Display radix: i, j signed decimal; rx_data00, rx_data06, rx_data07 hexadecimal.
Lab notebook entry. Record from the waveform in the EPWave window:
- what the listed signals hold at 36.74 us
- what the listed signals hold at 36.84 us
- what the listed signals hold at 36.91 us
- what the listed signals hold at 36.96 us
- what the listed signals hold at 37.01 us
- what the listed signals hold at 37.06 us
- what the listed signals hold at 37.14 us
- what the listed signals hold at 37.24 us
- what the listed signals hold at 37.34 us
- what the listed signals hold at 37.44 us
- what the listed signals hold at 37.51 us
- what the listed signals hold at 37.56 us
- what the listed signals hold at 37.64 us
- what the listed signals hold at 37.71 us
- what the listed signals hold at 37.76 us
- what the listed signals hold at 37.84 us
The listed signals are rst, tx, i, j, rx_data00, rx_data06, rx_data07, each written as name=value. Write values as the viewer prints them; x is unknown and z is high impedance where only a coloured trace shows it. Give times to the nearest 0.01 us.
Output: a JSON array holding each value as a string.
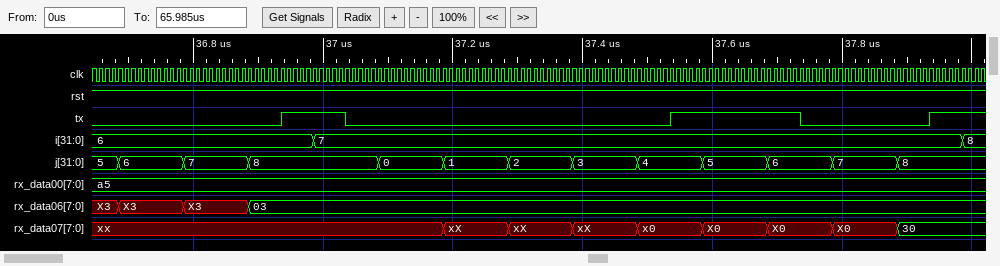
["rst=1, tx=0, i=6, j=6, rx_data00=a5, rx_data06=X3, rx_data07=xx", "rst=1, tx=0, i=6, j=7, rx_data00=a5, rx_data06=X3, rx_data07=xx", "rst=1, tx=0, i=6, j=8, rx_data00=a5, rx_data06=03, rx_data07=xx", "rst=1, tx=1, i=6, j=8, rx_data00=a5, rx_data06=03, rx_data07=xx", "rst=1, tx=1, i=7, j=8, rx_data00=a5, rx_data06=03, rx_data07=xx", "rst=1, tx=0, i=7, j=8, rx_data00=a5, rx_data06=03, rx_data07=xx", "rst=1, tx=0, i=7, j=0, rx_data00=a5, rx_data06=03, rx_data07=xx", "rst=1, tx=0, i=7, j=1, rx_data00=a5, rx_data06=03, rx_data07=xX", "rst=1, tx=0, i=7, j=2, rx_data00=a5, rx_data06=03, rx_data07=xX", "rst=1, tx=0, i=7, j=3, rx_data00=a5, rx_data06=03, rx_data07=xX", "rst=1, tx=0, i=7, j=4, rx_data00=a5, rx_data06=03, rx_data07=x0", "rst=1, tx=1, i=7, j=4, rx_data00=a5, rx_data06=03, rx_data07=x0", "rst=1, tx=1, i=7, j=5, rx_data00=a5, rx_data06=03, rx_data07=X0", "rst=1, tx=1, i=7, j=6, rx_data00=a5, rx_data06=03, rx_data07=X0", "rst=1, tx=0, i=7, j=6, rx_data00=a5, rx_data06=03, rx_data07=X0", "rst=1, tx=0, i=7, j=7, rx_data00=a5, rx_data06=03, rx_data07=X0"]
